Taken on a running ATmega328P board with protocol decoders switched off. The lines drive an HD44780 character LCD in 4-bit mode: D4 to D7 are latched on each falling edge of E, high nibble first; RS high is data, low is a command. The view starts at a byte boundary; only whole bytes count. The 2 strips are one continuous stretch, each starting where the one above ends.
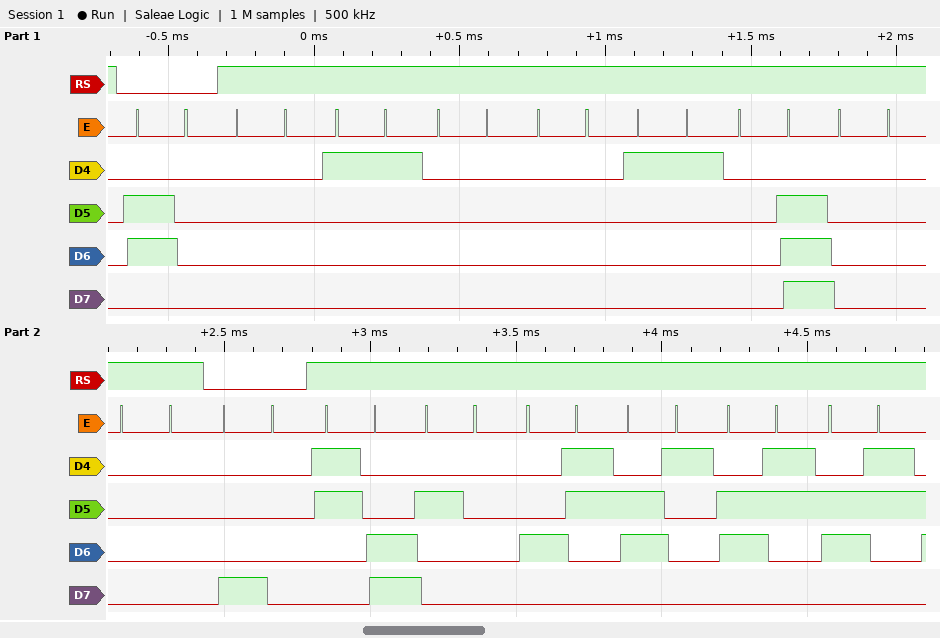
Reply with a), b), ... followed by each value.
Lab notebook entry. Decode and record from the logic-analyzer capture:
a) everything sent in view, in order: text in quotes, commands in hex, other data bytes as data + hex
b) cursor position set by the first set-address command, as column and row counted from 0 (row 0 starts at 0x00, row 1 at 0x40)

a) 0x60 data 00 11 00 00 11 0E 00 00 0x80 "< Cacc"
b) column 0, row 0
